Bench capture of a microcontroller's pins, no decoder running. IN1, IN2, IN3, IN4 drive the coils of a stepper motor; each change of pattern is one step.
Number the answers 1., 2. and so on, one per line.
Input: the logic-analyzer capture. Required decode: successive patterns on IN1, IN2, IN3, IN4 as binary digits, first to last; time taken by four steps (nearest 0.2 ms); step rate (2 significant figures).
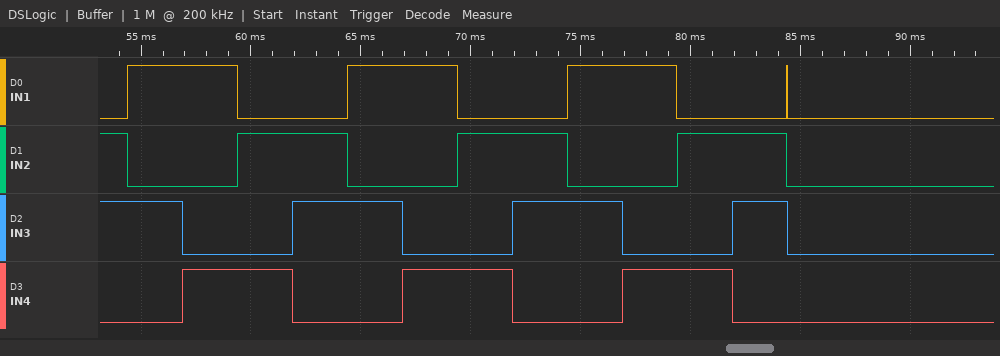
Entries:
1. 0110 1010 1001 0101 0110 1010 1001 0101 0110 1010 1001 0101 0110 0000
2. 10.0 ms
3. 400 steps/s
